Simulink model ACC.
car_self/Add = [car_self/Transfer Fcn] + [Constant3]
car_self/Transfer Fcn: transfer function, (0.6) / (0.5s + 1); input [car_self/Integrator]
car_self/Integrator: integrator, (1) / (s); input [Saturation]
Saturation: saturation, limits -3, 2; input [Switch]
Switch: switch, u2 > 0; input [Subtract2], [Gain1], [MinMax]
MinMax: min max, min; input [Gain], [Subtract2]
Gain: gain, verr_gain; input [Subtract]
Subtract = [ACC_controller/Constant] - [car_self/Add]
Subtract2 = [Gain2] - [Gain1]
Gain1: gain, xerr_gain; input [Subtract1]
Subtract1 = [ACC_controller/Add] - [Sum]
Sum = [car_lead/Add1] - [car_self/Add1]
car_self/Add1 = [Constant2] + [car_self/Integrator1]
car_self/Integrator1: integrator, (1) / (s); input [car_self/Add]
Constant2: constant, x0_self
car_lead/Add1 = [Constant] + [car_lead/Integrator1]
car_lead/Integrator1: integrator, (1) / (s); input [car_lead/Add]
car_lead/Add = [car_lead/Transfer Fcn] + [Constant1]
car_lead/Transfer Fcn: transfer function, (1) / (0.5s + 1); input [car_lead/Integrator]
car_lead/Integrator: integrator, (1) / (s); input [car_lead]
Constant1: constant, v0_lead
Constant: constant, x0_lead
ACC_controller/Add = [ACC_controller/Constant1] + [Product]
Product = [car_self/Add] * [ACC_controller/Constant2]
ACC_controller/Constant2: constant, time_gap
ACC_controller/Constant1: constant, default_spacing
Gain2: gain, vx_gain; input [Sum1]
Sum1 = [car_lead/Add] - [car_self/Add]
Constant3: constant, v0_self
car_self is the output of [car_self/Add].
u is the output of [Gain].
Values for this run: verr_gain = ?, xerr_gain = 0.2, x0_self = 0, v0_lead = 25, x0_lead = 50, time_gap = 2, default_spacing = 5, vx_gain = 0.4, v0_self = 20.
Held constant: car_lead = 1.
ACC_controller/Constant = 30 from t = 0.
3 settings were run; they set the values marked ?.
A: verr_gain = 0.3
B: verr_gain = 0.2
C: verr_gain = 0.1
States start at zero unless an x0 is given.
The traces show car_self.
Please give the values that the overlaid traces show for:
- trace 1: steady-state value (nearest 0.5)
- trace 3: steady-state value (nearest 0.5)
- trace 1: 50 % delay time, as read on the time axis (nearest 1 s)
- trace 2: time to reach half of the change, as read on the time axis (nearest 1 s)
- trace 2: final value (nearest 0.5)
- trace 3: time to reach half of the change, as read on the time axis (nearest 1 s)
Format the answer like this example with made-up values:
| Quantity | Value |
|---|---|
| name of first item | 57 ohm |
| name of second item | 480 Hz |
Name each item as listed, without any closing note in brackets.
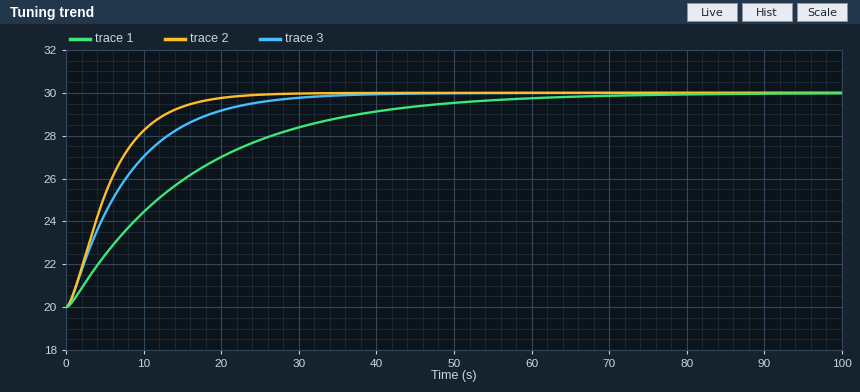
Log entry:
| Quantity | Value |
|---|---|
| trace 1: steady-state value | 30.0 |
| trace 3: steady-state value | 30.0 |
| trace 1: 50 % delay time, as read on the time axis | 12 s |
| trace 2: time to reach half of the change, as read on the time axis | 5 s |
| trace 2: final value | 30.0 |
| trace 3: time to reach half of the change, as read on the time axis | 6 s |
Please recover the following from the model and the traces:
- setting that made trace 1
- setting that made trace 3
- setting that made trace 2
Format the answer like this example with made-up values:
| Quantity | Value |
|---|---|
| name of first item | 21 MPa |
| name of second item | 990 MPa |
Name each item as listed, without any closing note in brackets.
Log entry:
| Quantity | Value |
|---|---|
| setting that made trace 1 | C |
| setting that made trace 3 | B |
| setting that made trace 2 | A |
